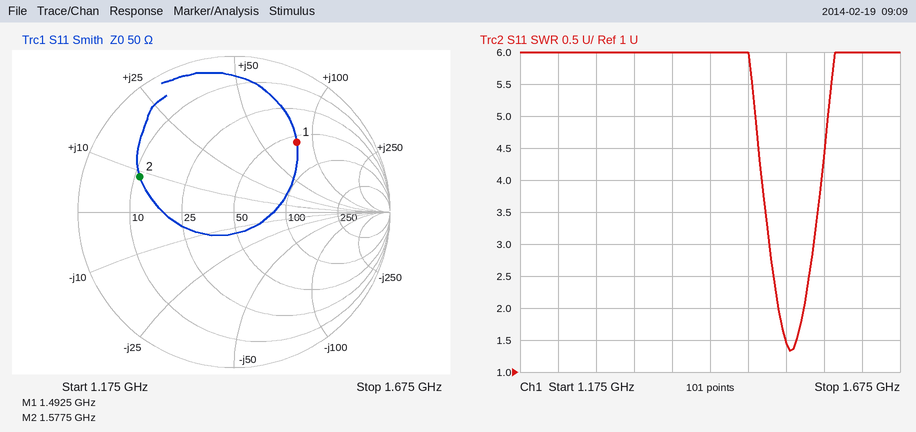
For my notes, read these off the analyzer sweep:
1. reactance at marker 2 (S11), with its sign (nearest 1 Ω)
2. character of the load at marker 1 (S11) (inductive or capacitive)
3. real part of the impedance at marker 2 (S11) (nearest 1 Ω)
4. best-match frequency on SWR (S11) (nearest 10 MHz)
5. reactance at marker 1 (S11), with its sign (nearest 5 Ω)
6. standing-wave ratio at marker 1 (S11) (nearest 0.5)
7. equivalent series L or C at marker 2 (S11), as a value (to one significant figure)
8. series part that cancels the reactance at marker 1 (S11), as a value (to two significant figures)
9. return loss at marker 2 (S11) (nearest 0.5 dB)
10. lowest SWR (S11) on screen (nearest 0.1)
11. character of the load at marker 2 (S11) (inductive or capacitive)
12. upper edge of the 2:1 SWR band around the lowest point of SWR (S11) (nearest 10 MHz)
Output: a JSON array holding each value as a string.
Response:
["+9 Ω", "inductive", "11 Ω", "1.53 GHz", "+80 Ω", "4.0", "900 pH", "1.3 pF", "4.0 dB", "1.3", "inductive", "1.55 GHz"]
